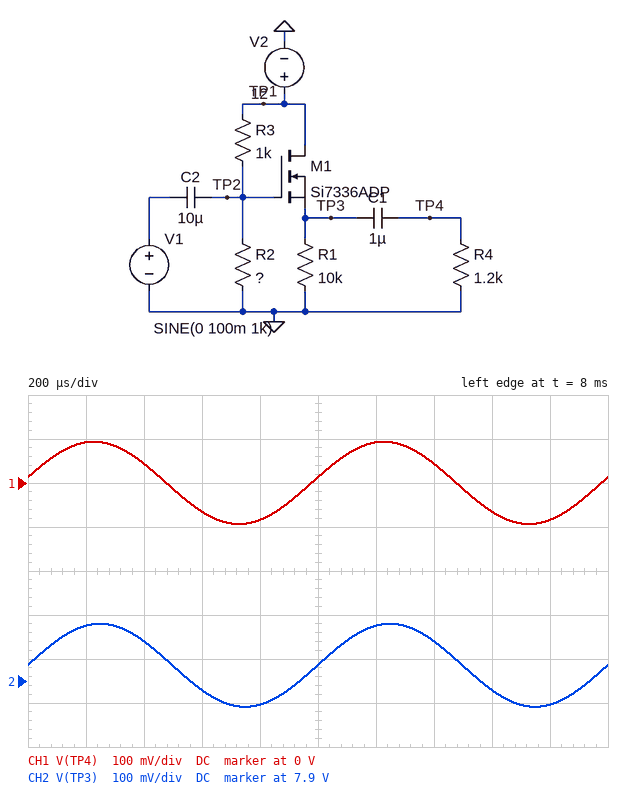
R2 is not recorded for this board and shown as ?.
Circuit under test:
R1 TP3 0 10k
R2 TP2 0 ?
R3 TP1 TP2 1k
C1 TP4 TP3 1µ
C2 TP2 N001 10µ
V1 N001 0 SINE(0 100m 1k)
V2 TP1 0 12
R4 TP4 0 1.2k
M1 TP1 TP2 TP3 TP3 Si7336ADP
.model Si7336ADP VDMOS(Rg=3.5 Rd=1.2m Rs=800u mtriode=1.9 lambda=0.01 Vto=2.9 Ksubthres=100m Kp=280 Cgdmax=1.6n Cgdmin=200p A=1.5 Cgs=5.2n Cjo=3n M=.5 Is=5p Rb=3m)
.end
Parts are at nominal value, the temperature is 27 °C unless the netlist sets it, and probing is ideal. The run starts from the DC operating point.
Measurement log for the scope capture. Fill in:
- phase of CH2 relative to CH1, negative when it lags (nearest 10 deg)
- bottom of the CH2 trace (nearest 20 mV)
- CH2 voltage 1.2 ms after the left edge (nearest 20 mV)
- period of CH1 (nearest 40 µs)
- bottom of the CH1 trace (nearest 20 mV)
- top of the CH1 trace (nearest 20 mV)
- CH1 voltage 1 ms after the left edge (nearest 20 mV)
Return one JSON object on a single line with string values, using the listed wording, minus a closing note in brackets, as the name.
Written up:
{"phase of CH2 relative to CH1, negative when it lags": "-10 deg", "bottom of the CH2 trace": "7.84 V", "CH2 voltage 1.2 ms after the left edge": "8.02 V", "period of CH1": "1.00 ms", "bottom of the CH1 trace": "-100 mV", "top of the CH1 trace": "100 mV", "CH1 voltage 1 ms after the left edge": "20 mV"}
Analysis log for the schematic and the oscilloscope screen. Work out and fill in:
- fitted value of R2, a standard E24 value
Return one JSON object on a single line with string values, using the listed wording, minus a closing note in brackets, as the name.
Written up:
{"fitted value of R2, a standard E24 value": "6.8 kΩ"}
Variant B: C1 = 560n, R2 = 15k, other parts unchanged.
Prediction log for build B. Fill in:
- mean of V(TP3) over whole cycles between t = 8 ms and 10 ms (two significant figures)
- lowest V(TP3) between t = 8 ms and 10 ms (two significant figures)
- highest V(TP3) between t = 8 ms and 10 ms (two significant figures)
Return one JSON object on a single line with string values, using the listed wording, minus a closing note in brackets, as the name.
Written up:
{"mean of V(TP3) over whole cycles between t = 8 ms and 10 ms": "8.7 V", "lowest V(TP3) between t = 8 ms and 10 ms": "8.6 V", "highest V(TP3) between t = 8 ms and 10 ms": "8.8 V"}
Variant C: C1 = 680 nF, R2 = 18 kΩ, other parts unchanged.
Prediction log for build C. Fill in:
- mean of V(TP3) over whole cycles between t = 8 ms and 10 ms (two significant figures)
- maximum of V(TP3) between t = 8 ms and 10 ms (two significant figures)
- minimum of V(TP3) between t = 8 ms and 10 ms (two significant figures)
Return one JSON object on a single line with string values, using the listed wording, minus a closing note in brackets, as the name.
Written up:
{"mean of V(TP3) over whole cycles between t = 8 ms and 10 ms": "8.8 V", "maximum of V(TP3) between t = 8 ms and 10 ms": "8.9 V", "minimum of V(TP3) between t = 8 ms and 10 ms": "8.7 V"}
